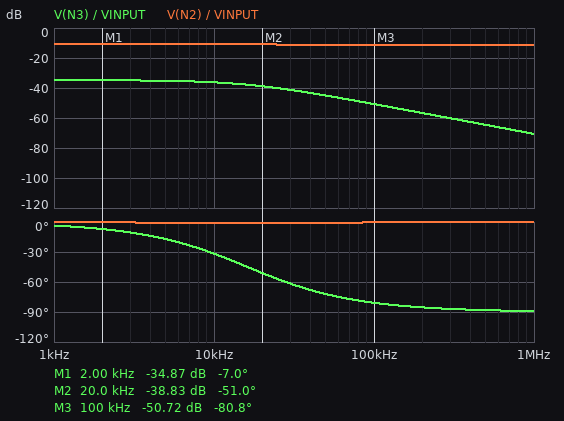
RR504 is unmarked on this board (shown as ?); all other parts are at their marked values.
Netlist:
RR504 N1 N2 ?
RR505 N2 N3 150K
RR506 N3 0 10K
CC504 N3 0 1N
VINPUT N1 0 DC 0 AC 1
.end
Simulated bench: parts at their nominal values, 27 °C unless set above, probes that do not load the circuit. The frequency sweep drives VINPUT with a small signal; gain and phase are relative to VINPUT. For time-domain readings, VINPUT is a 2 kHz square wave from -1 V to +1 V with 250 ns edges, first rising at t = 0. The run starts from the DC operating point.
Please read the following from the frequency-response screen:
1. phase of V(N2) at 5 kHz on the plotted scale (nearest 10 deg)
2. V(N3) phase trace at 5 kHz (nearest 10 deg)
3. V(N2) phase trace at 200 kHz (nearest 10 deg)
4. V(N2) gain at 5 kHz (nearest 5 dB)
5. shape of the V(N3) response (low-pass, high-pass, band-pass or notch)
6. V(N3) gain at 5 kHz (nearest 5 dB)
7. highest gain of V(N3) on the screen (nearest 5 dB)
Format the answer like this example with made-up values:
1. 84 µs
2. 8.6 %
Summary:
1. 0 deg
2. -20 deg
3. 0 deg
4. -10 dB
5. low-pass
6. -35 dB
7. -35 dB
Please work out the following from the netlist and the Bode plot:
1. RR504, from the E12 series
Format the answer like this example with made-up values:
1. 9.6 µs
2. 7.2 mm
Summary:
1. 390 kΩ
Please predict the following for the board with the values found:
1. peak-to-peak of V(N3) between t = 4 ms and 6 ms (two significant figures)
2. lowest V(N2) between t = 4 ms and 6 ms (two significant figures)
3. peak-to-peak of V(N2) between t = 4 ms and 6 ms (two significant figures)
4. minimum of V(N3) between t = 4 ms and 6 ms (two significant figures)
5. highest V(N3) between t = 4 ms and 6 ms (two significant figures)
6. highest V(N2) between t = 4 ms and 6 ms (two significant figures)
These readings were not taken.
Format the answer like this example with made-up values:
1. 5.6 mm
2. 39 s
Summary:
1. 36 mV
2. -290 mV
3. 580 mV
4. -18 mV
5. 18 mV
6. 290 mV
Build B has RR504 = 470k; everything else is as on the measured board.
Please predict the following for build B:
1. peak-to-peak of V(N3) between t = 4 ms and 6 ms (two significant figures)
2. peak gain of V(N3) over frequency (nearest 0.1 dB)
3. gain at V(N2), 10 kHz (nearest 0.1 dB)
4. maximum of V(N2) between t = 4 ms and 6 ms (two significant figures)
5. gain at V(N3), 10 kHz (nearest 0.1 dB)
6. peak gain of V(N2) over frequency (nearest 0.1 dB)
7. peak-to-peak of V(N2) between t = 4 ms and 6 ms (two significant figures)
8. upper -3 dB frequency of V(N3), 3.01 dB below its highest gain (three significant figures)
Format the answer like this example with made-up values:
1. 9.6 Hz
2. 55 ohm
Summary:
1. 32 mV
2. -36.0 dB
3. -12.0 dB
4. 250 mV
5. -37.4 dB
6. -11.9 dB
7. 510 mV
8. 16.2 kHz
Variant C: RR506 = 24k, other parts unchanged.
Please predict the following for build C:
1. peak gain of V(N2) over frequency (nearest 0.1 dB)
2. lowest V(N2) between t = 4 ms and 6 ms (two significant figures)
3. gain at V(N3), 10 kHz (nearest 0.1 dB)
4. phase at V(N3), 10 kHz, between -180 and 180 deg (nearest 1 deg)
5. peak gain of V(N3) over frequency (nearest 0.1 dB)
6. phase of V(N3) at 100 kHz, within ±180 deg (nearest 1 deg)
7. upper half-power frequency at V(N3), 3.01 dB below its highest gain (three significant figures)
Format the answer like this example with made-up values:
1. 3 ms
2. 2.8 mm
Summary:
1. -10.2 dB
2. -310 mV
3. -32.3 dB
4. -55 deg
5. -27.4 dB
6. -86 deg
7. 6.93 kHz
